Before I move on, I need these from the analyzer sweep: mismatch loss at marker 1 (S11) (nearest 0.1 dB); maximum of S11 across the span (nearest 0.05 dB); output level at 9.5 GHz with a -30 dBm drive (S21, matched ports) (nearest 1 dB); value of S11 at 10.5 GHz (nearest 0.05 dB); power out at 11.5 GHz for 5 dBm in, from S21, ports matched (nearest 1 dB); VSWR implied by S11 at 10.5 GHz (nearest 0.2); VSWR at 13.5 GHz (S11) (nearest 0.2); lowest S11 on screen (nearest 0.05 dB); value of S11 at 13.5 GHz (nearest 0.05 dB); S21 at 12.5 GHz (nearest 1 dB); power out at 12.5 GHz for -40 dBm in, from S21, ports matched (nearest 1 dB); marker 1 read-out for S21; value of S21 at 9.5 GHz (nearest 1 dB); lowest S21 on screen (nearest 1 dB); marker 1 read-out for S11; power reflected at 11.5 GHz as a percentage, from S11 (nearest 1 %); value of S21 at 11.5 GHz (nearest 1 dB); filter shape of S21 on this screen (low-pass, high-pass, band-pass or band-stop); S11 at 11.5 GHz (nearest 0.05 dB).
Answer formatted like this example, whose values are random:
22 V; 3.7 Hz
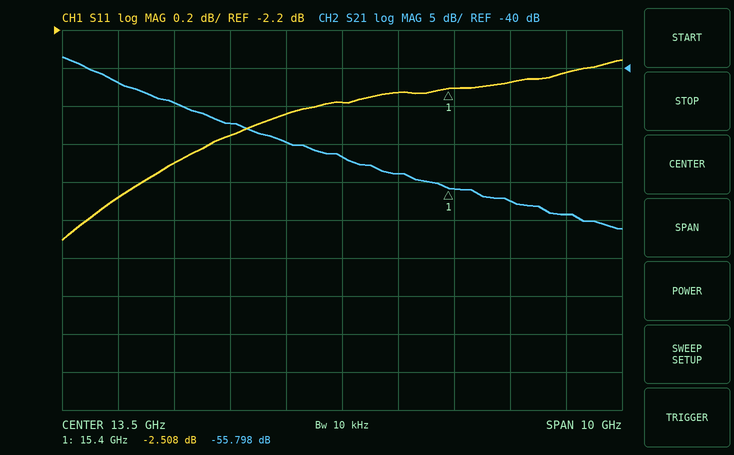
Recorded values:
3.6 dB; -2.35 dB; -72 dBm; -2.90 dB; -42 dBm; 6.0; 6.8; -3.30 dB; -2.60 dB; -50 dB; -90 dBm; -55.798 dB; -42 dB; -61 dB; -2.508 dB; 53 %; -47 dB; low-pass; -2.75 dB
